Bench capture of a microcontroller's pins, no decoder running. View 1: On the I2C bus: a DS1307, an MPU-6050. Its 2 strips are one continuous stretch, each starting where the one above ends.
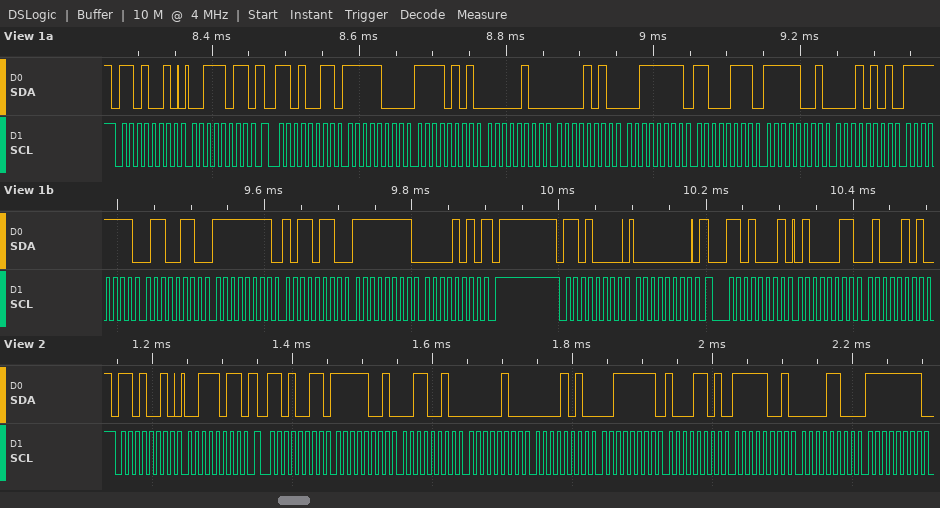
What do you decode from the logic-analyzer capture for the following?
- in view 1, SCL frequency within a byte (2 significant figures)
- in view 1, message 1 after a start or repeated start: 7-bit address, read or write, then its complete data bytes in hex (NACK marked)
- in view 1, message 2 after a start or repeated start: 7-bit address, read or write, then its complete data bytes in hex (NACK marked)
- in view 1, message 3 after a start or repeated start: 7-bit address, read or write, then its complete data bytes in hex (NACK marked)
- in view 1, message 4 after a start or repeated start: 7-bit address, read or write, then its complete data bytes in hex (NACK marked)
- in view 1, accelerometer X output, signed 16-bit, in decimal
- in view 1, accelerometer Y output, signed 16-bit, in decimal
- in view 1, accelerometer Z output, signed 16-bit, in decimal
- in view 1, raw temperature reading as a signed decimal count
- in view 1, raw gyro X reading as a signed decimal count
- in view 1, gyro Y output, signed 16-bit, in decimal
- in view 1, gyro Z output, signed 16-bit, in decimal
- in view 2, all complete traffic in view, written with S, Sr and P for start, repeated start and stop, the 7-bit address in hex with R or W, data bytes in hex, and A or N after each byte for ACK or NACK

100 kHz
0x69 write: 3B
0x69 read: F8 F5 04 0A 3F C7 F9 15 FF 66 FF B6 FF 0A NACK
0x68 write: 00
0x68 read: 43 45
-1803
1034
16327
-1771
-154
-74
-246
S 69W A 3B A Sr 69R A F9 A 32 A 04 A 0A A 3F A 8D A F9 A 0C A FF A
